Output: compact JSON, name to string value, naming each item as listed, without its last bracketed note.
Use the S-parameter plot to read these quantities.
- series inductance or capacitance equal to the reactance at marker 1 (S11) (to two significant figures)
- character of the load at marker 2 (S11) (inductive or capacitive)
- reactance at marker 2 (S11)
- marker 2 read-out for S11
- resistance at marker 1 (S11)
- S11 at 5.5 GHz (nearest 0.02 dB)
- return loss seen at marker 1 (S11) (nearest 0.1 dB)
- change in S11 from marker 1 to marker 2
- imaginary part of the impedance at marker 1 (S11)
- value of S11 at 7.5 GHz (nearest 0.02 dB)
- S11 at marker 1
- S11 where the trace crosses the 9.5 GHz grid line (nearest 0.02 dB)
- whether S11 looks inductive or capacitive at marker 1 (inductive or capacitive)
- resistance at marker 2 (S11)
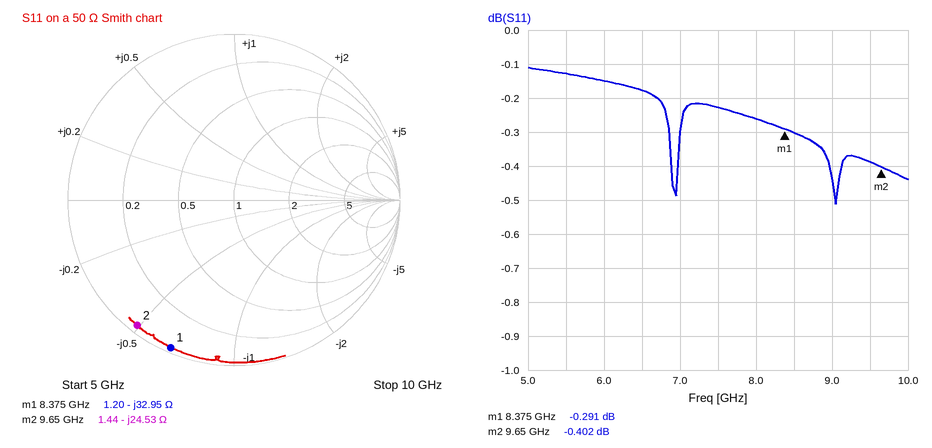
{"series inductance or capacitance equal to the reactance at marker 1 (S11)": "580 fF", "character of the load at marker 2 (S11)": "capacitive", "reactance at marker 2": "-24.53 Ω", "marker 2 read-out for S11": "-0.402 dB", "resistance at marker 1": "1.20 Ω", "S11 at 5.5 GHz": "-0.12 dB", "return loss seen at marker 1 (S11)": "0.3 dB", "change in S11 from marker 1 to marker 2": "-0.111 dB", "imaginary part of the impedance at marker 1": "-32.95 Ω", "value of S11 at 7.5 GHz": "-0.22 dB", "S11 at marker 1": "-0.291 dB", "S11 where the trace crosses the 9.5 GHz grid line": "-0.38 dB", "whether S11 looks inductive or capacitive at marker 1": "capacitive", "resistance at marker 2": "1.44 Ω"}
